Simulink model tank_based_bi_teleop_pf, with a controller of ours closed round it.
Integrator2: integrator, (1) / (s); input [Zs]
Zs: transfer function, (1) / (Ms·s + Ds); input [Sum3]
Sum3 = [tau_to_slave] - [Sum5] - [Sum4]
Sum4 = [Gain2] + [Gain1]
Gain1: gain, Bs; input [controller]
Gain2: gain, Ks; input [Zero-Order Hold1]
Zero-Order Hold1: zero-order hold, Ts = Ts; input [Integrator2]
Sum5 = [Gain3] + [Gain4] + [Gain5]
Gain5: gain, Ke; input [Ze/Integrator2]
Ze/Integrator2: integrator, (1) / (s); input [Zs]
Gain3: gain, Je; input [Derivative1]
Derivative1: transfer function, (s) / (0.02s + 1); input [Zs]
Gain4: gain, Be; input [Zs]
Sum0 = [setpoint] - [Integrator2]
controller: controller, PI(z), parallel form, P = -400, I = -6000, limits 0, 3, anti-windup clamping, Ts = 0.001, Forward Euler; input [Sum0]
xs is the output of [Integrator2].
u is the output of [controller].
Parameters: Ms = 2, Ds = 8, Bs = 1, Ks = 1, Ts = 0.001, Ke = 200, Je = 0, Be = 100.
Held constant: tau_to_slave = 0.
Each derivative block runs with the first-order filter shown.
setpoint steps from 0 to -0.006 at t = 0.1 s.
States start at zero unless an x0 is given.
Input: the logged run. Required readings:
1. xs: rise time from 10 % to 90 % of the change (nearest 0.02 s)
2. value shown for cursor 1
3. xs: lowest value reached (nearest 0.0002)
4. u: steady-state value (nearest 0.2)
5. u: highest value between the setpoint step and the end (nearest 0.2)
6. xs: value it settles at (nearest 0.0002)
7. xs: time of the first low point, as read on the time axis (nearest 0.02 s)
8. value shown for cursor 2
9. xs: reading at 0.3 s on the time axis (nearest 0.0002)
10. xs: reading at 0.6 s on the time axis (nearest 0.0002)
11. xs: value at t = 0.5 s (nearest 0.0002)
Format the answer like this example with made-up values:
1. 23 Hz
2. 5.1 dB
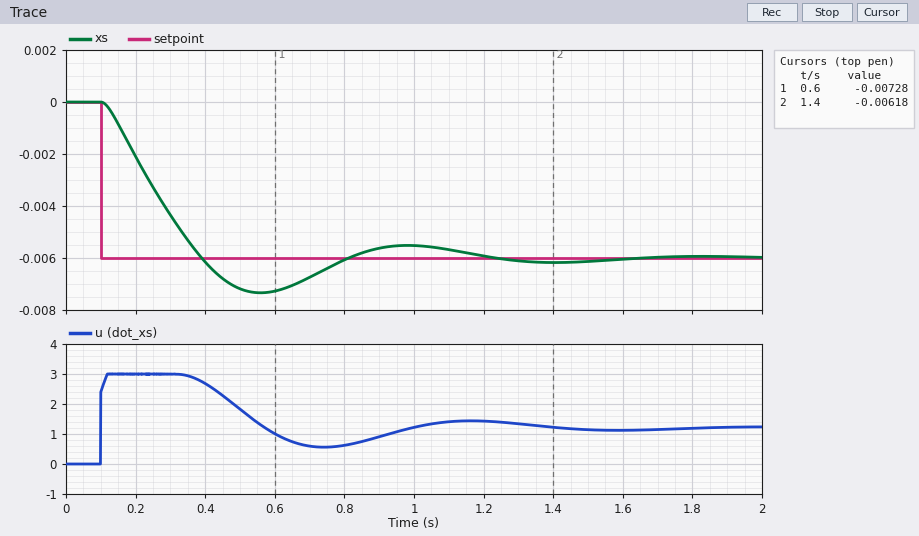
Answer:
1. 0.22 s
2. -0.00728
3. -0.0074
4. 1.2
5. 3.0
6. -0.0060
7. 0.56 s
8. -0.00618
9. -0.0044
10. -0.0072
11. -0.0072
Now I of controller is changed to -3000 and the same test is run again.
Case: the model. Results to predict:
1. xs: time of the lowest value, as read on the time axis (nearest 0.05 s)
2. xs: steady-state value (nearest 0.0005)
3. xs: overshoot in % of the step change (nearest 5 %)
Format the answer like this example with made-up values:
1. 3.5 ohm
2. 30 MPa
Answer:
1. 0.60 s
2. -0.0060
3. 20 %
